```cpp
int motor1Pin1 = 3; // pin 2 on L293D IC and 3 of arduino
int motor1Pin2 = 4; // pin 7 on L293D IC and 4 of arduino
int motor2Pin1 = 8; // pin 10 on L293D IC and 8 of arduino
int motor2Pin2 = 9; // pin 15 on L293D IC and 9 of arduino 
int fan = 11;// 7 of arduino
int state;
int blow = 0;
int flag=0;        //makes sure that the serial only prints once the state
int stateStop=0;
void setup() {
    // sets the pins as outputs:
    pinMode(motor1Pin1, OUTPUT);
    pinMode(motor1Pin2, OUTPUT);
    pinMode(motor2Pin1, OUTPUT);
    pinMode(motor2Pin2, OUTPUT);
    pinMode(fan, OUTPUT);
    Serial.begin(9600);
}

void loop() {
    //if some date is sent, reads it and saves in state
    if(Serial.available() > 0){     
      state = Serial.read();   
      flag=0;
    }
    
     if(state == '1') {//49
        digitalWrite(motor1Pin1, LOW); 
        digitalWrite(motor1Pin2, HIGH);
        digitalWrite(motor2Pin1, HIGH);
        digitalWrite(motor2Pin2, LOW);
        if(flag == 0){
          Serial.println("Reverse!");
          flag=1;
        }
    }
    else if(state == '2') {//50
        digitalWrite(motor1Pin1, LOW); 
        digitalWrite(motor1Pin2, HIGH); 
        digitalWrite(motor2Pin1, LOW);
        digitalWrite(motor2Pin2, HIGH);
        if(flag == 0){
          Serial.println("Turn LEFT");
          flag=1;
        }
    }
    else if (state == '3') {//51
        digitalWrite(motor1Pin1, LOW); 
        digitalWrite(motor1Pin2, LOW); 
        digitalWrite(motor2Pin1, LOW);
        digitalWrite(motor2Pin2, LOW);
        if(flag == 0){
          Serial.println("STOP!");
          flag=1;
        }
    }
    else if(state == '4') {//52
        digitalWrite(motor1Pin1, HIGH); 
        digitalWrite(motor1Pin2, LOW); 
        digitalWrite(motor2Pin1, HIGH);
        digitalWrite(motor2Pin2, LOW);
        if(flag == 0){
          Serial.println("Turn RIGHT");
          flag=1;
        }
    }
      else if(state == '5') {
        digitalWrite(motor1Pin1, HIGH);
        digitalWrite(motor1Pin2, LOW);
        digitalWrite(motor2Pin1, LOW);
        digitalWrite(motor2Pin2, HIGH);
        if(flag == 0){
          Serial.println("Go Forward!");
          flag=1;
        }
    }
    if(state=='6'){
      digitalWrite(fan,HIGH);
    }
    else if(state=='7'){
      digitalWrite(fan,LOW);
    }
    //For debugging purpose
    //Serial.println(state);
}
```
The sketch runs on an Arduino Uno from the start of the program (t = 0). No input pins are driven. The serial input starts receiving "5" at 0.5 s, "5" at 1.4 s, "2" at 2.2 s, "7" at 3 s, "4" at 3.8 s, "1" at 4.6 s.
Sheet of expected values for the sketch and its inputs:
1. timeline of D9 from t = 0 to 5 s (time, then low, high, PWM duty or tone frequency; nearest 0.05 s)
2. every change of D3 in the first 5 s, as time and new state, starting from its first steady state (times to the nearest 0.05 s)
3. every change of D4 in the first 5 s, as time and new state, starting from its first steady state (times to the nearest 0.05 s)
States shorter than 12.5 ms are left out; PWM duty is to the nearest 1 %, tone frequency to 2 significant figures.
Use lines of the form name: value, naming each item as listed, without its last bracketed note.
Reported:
timeline of D9 from t = 0 to 5 s: 0 s low; 0.5 s high; 3.8 s low
every change of D3 in the first 5 s, as time and new state, starting from its first steady state: 0 s low; 0.5 s high; 2.2 s low; 3.8 s high; 4.6 s low
every change of D4 in the first 5 s, as time and new state, starting from its first steady state: 0 s low; 2.2 s high; 3.8 s low; 4.6 s high
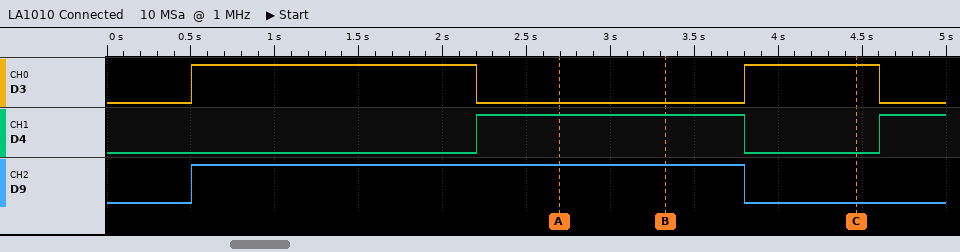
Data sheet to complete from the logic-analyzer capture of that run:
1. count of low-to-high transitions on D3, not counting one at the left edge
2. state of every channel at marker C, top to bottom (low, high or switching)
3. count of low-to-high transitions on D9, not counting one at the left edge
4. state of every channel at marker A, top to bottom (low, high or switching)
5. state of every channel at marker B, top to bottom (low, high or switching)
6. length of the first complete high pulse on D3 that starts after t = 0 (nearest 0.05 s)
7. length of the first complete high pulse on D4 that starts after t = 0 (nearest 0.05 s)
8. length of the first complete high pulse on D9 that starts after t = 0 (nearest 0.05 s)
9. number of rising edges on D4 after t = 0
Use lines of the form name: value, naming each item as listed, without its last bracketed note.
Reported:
count of low-to-high transitions on D3, not counting one at the left edge: 2
state of every channel at marker C, top to bottom: D3 high, D4 low, D9 low
count of low-to-high transitions on D9, not counting one at the left edge: 1
state of every channel at marker A, top to bottom: D3 low, D4 high, D9 high
state of every channel at marker B, top to bottom: D3 low, D4 high, D9 high
length of the first complete high pulse on D3 that starts after t = 0: 1.70 s
length of the first complete high pulse on D4 that starts after t = 0: 1.60 s
length of the first complete high pulse on D9 that starts after t = 0: 3.30 s
number of rising edges on D4 after t = 0: 2
